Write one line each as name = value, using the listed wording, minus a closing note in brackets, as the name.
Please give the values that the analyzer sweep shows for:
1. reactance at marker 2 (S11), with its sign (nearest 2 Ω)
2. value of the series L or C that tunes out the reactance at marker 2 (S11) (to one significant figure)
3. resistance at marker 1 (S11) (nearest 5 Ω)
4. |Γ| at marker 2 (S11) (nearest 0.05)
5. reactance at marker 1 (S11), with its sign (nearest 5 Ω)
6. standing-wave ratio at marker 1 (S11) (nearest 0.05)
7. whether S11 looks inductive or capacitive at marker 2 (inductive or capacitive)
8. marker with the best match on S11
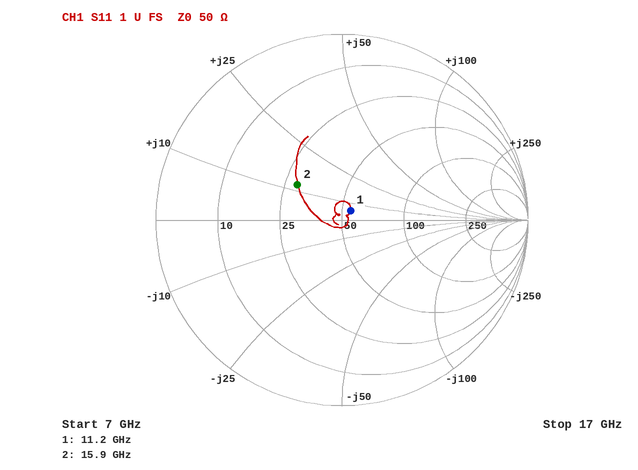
reactance at marker 2 (S11), with its sign = +12 Ω
value of the series L or C that tunes out the reactance at marker 2 (S11) = 800 fF
resistance at marker 1 (S11) = 55 Ω
|Γ| at marker 2 (S11) = 0.30
reactance at marker 1 (S11), with its sign = +5 Ω
standing-wave ratio at marker 1 (S11) = 1.15
whether S11 looks inductive or capacitive at marker 2 = inductive
marker with the best match on S11 = marker 1
